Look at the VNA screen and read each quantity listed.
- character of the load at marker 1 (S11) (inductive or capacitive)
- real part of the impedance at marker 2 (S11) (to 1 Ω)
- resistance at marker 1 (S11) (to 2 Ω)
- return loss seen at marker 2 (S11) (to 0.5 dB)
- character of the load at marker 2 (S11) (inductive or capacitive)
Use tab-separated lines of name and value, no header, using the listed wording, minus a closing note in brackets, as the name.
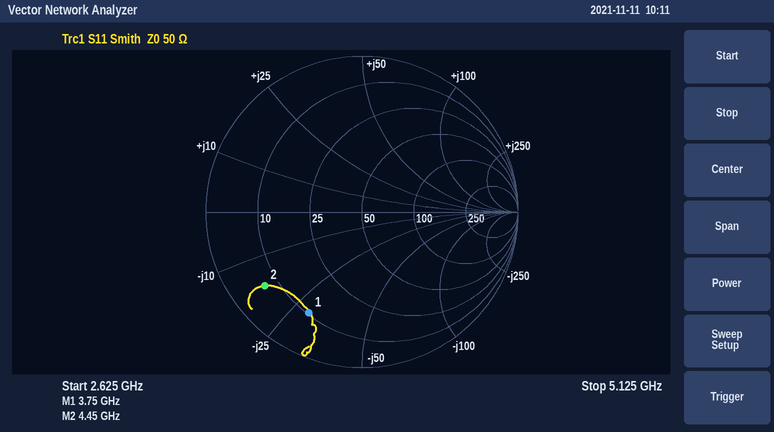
character of the load at marker 1 (S11)	capacitive
real part of the impedance at marker 2 (S11)	7 Ω
resistance at marker 1 (S11)	10 Ω
return loss seen at marker 2 (S11)	2.0 dB
character of the load at marker 2 (S11)	capacitive
